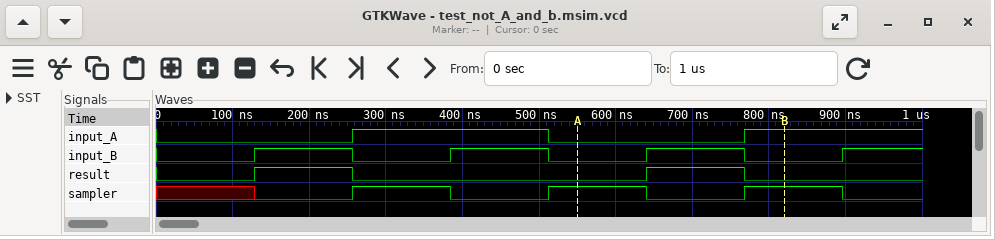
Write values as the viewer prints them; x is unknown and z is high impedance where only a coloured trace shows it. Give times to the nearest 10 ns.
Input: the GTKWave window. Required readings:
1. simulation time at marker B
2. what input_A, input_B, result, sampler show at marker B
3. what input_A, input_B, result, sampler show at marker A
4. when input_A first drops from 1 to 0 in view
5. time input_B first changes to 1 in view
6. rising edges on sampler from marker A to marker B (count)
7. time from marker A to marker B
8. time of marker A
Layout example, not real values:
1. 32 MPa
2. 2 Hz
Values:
1. 820 ns
2. input_A=1, input_B=0, result=0, sampler=1
3. input_A=0, input_B=0, result=0, sampler=1
4. 510 ns
5. 130 ns
6. 1
7. 270 ns
8. 550 ns
